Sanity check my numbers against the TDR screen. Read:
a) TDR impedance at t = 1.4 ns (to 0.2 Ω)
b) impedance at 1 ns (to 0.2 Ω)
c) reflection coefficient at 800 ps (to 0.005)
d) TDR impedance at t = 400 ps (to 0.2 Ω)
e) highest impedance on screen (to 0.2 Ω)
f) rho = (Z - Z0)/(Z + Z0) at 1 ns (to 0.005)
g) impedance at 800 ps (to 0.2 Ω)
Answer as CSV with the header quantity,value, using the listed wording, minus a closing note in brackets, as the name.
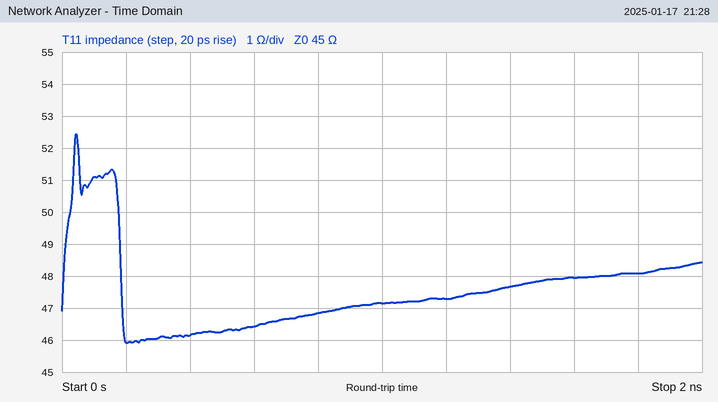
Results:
quantity,value
TDR impedance at t = 1.4 ns,47.6 Ω
impedance at 1 ns,47.2 Ω
reflection coefficient at 800 ps,+0.020
TDR impedance at t = 400 ps,46.2 Ω
highest impedance on screen,52.4 Ω
rho = (Z - Z0)/(Z + Z0) at 1 ns,+0.025
impedance at 800 ps,46.8 Ω
